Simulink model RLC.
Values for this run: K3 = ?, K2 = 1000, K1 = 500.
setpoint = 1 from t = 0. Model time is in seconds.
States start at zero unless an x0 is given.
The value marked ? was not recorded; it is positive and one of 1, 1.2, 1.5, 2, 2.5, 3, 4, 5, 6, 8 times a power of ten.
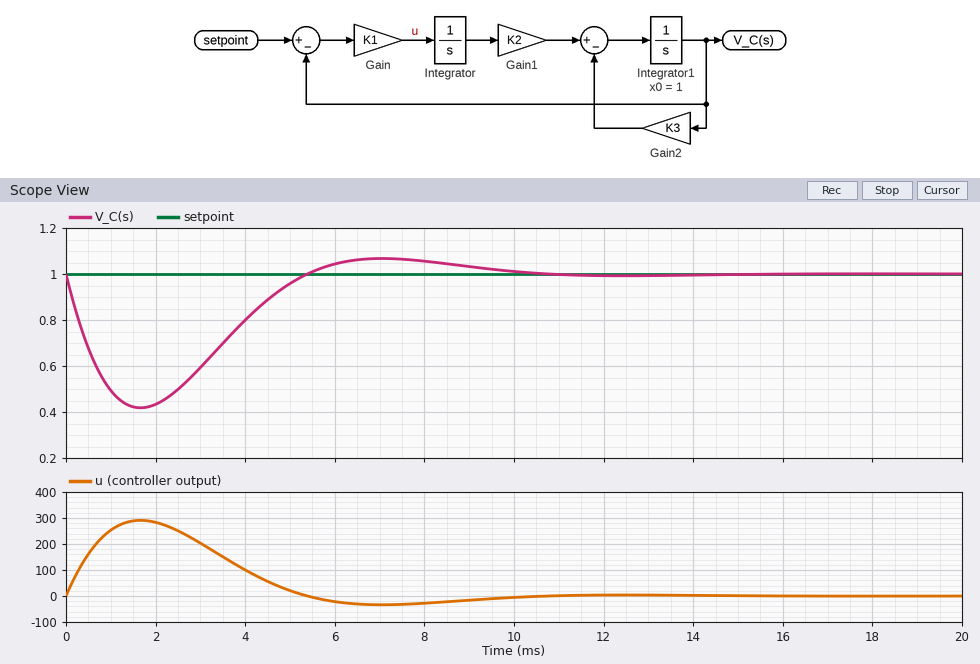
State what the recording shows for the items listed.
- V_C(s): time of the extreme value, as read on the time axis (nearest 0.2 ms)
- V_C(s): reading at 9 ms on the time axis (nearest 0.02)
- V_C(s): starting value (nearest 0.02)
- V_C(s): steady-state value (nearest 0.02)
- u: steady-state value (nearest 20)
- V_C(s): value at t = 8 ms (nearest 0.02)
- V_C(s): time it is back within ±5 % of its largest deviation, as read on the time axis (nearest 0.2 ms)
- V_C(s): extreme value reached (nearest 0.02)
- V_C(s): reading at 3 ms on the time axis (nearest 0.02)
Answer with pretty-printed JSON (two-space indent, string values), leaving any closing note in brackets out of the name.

{
  "V_C(s): time of the extreme value, as read on the time axis": "1.6 ms",
  "V_C(s): reading at 9 ms on the time axis": "1.04",
  "V_C(s): starting value": "1.00",
  "V_C(s): steady-state value": "1.00",
  "u: steady-state value": "0",
  "V_C(s): value at t = 8 ms": "1.06",
  "V_C(s): time it is back within ±5 % of its largest deviation, as read on the time axis": "9.2 ms",
  "V_C(s): extreme value reached": "0.42",
  "V_C(s): reading at 3 ms on the time axis": "0.60"
}
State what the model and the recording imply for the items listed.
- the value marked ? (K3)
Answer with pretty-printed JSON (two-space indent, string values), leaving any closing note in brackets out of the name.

{
  "the value marked ?": "800"
}
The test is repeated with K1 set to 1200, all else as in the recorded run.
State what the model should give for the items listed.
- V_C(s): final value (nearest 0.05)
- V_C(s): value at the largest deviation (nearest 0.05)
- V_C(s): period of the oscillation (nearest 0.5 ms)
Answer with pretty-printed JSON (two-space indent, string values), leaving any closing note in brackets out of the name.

{
  "V_C(s): final value": "1.00",
  "V_C(s): value at the largest deviation": "0.55",
  "V_C(s): period of the oscillation": "6.0 ms"
}
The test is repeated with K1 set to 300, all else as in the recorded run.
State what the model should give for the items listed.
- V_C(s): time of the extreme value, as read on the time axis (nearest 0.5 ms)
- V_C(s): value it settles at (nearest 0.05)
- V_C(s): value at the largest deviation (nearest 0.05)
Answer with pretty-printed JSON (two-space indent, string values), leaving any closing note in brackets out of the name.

{
  "V_C(s): time of the extreme value, as read on the time axis": "2.0 ms",
  "V_C(s): value it settles at": "1.00",
  "V_C(s): value at the largest deviation": "0.35"
}
